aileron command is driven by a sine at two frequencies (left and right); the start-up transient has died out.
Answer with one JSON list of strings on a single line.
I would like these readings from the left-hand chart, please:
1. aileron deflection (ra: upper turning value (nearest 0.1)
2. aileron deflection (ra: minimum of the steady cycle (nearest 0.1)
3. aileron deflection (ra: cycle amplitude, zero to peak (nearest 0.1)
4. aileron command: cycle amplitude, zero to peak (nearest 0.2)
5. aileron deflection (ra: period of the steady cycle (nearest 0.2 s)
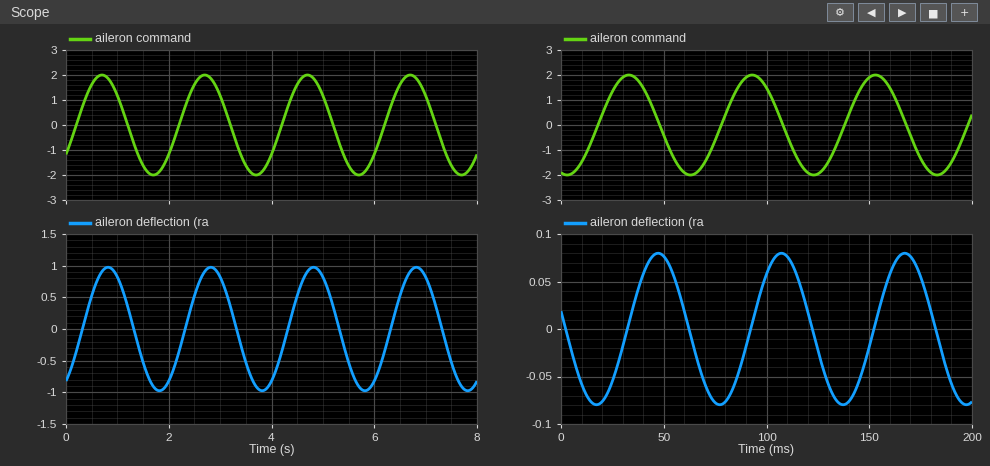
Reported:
["1.0", "-1.0", "1.0", "2.0", "2.0 s"]
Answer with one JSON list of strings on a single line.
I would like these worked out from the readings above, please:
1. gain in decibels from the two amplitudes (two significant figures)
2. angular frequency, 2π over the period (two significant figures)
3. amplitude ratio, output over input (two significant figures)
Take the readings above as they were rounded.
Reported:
["-6.0 dB", "3.1 rad/s", "0.50"]
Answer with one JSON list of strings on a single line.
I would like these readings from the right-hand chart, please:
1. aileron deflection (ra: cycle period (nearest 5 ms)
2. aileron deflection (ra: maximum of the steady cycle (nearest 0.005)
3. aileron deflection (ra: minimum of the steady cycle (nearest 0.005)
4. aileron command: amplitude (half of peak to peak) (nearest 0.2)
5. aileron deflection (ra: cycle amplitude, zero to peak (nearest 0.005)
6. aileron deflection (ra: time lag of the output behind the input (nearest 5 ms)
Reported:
["60 ms", "0.080", "-0.080", "2.0", "0.080", "15 ms"]
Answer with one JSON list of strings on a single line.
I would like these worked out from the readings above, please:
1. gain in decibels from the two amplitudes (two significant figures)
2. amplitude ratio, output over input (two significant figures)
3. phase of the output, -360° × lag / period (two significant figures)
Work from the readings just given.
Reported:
["-28 dB", "0.040", "-90°"]
